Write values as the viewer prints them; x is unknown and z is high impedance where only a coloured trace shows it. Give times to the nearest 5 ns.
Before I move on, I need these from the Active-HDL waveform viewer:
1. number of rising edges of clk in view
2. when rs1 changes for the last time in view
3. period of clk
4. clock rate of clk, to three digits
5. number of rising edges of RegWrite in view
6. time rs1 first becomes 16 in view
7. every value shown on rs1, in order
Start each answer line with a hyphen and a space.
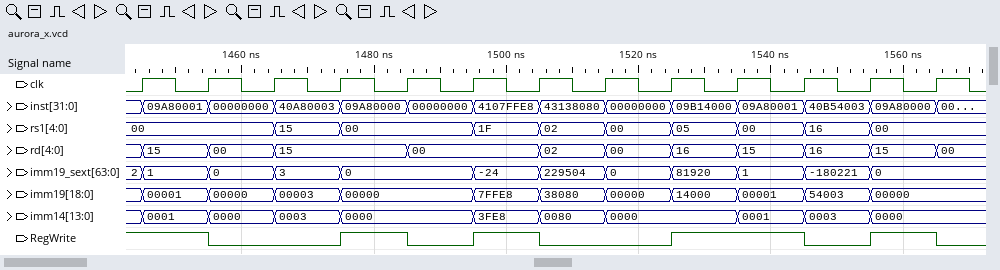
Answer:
- 13
- 1555 ns
- 10 ns
- 100 MHz
- 4
- 1545 ns
- 00, 15, 00, 1F, 02, 00, 05, 00, 16, 00
